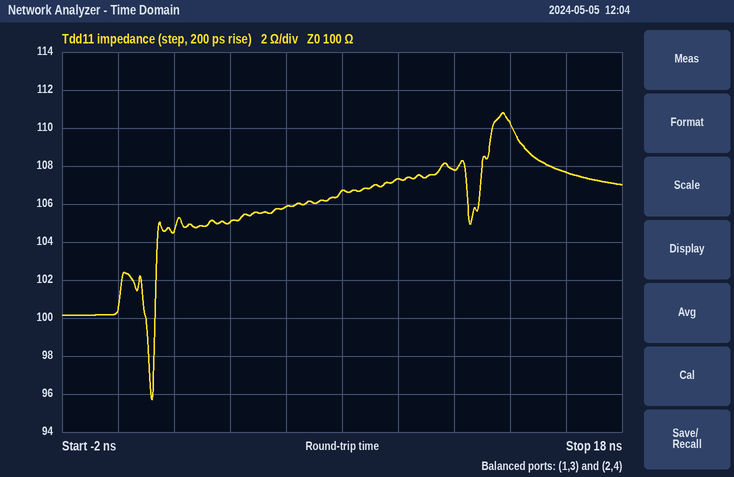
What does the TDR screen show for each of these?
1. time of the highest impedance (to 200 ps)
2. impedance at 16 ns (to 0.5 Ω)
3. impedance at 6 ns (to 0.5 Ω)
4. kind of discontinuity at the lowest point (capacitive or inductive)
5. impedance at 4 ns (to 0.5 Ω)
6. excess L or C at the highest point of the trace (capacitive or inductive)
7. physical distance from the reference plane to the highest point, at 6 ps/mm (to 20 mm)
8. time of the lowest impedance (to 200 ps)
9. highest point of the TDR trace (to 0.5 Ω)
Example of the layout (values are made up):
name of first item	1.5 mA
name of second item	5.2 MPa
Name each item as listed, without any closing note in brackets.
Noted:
time of the highest impedance	13.8 ns
impedance at 16 ns	107.5 Ω
impedance at 6 ns	106.0 Ω
kind of discontinuity at the lowest point	capacitive
impedance at 4 ns	105.0 Ω
excess L or C at the highest point of the trace	inductive
physical distance from the reference plane to the highest point, at 6 ps/mm	1.14 m
time of the lowest impedance	1.2 ns
highest point of the TDR trace	111.0 Ω
